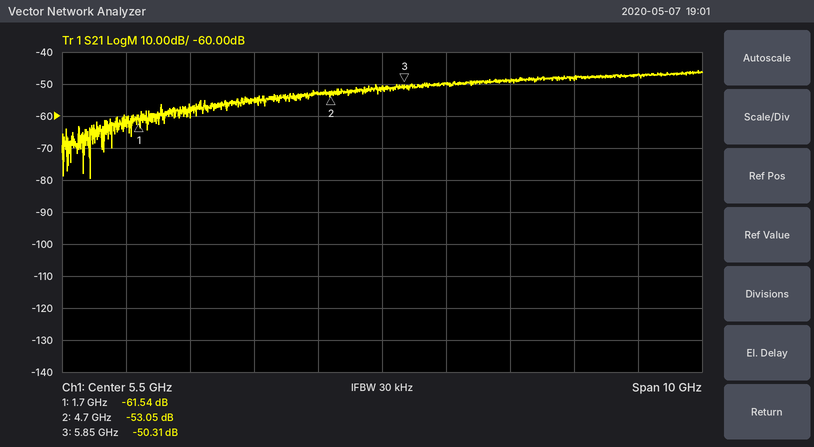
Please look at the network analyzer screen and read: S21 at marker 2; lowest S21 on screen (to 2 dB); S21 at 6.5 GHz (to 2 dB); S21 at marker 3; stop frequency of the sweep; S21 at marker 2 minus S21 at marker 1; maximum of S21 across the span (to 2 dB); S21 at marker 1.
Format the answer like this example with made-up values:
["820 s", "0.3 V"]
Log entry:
["-53.05 dB", "-80 dB", "-50 dB", "-50.31 dB", "10.5 GHz", "8.49 dB", "-46 dB", "-61.54 dB"]
